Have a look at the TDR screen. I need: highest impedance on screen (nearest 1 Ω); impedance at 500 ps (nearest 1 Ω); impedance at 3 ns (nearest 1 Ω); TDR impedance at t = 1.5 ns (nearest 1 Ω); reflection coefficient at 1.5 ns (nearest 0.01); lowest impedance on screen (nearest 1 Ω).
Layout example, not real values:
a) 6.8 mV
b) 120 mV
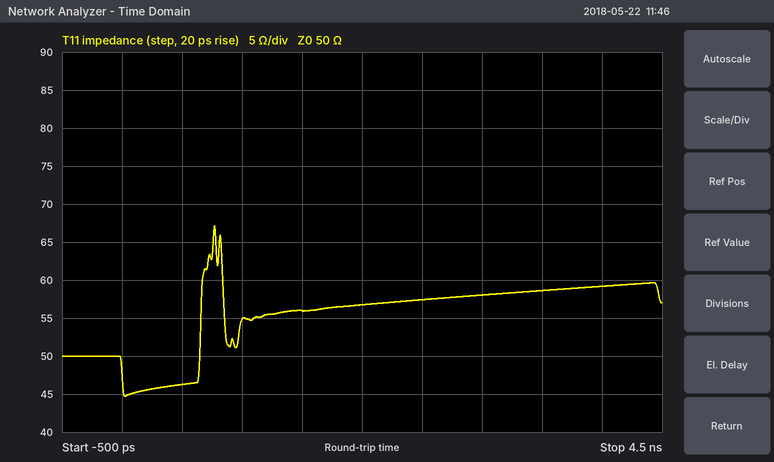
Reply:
a) 67 Ω
b) 46 Ω
c) 58 Ω
d) 56 Ω
e) +0.06
f) 45 Ω
